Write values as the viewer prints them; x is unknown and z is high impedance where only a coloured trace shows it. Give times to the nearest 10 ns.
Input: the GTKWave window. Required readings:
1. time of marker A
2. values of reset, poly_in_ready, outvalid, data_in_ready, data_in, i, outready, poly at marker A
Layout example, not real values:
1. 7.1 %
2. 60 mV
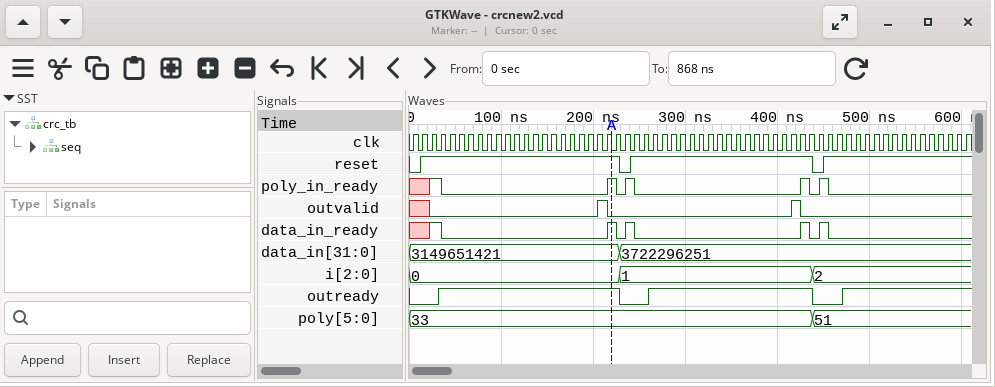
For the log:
1. 220 ns
2. reset=1, poly_in_ready=1, outvalid=0, data_in_ready=1, data_in=3149651421, i=0, outready=1, poly=33
